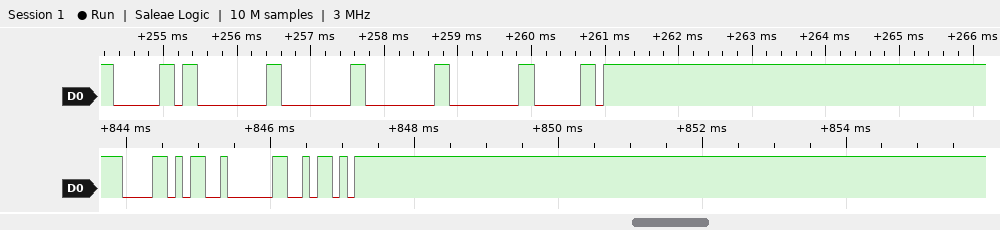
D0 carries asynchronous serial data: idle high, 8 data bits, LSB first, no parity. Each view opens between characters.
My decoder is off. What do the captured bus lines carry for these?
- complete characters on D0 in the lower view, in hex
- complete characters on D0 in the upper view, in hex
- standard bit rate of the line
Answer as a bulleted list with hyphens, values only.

- 58, 02, 5A
- 60, 00, 00, 00, 00, 60
- 9600 baud
